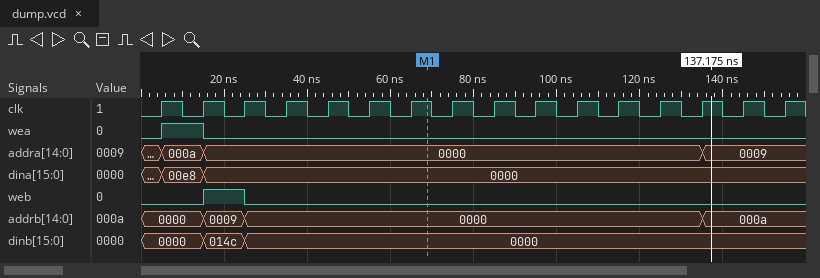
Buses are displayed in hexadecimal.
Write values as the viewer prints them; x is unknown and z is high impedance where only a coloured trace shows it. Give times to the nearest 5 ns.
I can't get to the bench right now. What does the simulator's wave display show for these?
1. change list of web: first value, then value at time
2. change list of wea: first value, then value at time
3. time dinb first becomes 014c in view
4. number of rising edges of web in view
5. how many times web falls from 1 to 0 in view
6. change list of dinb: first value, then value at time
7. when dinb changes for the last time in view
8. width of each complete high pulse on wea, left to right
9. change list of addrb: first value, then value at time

0, 1 at 15 ns, 0 at 25 ns
0, 1 at 5 ns, 0 at 15 ns
15 ns
1
1
0000, 014c at 15 ns, 0000 at 25 ns
25 ns
10 ns
0000, 0009 at 15 ns, 0000 at 25 ns, 000a at 135 ns
